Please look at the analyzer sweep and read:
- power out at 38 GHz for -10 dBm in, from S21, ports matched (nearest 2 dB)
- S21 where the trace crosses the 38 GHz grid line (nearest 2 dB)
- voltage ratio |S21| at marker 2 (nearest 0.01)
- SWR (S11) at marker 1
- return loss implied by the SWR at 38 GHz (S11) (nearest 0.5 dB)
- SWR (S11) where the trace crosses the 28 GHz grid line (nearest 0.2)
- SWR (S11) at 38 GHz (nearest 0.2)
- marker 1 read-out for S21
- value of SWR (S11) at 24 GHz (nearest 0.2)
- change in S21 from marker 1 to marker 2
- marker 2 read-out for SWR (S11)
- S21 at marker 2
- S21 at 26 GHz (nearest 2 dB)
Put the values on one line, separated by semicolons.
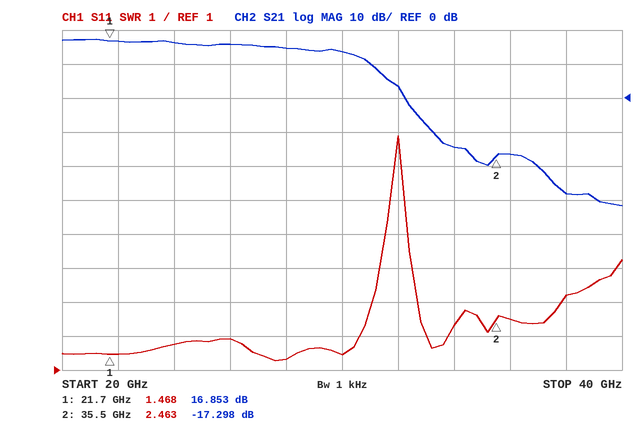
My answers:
-38 dBm; -28 dB; 0.14; 1.468; 5.5 dB; 1.4; 3.2; 16.853 dB; 1.8; -34.151 dB; 2.463; -17.298 dB; 16 dB
